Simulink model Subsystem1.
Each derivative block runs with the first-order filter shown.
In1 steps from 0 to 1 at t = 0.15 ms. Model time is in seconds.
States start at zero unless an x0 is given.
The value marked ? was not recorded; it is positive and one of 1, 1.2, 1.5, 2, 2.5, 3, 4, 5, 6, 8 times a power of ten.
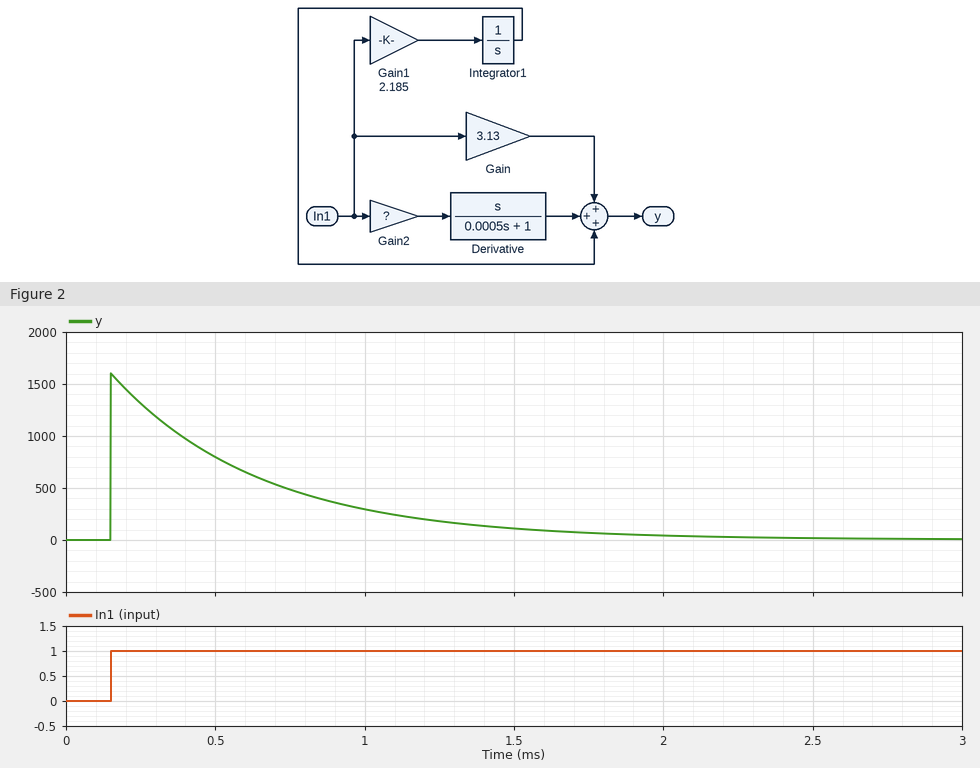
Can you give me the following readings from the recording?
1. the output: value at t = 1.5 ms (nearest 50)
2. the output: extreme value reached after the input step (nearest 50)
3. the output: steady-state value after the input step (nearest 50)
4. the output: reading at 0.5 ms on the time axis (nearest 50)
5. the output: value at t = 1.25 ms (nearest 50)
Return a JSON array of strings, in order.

["100", "1600", "0", "800", "200"]
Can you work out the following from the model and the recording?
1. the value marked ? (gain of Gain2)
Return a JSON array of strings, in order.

["0.8"]
